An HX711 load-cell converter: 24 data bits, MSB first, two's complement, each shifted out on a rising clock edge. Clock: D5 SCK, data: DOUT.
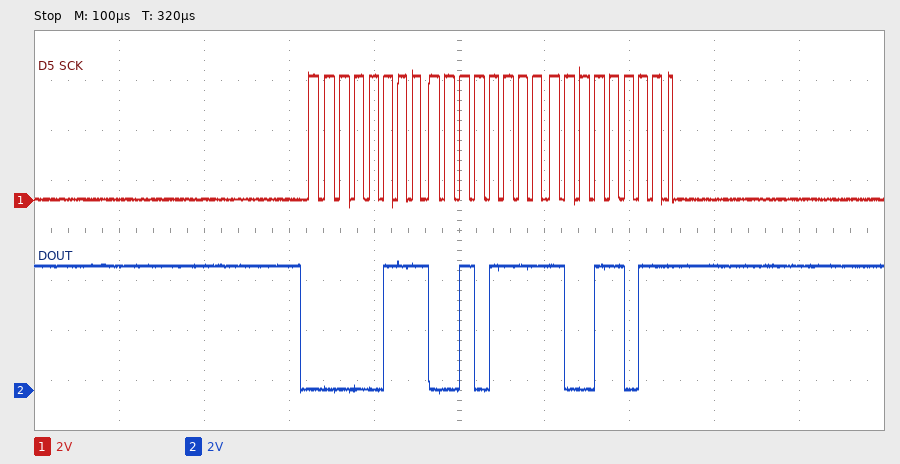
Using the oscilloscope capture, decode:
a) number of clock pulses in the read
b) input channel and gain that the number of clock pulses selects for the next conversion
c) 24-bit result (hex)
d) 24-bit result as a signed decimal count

25
channel A, gain 128
0x072F9B
470939
